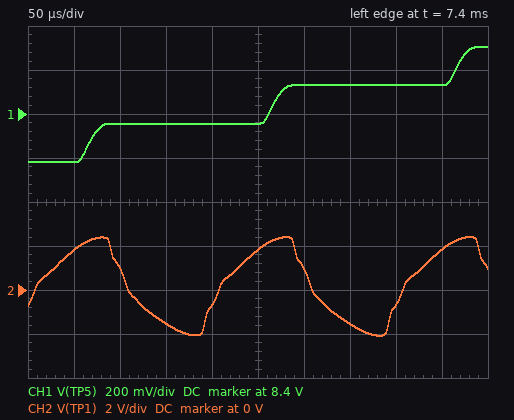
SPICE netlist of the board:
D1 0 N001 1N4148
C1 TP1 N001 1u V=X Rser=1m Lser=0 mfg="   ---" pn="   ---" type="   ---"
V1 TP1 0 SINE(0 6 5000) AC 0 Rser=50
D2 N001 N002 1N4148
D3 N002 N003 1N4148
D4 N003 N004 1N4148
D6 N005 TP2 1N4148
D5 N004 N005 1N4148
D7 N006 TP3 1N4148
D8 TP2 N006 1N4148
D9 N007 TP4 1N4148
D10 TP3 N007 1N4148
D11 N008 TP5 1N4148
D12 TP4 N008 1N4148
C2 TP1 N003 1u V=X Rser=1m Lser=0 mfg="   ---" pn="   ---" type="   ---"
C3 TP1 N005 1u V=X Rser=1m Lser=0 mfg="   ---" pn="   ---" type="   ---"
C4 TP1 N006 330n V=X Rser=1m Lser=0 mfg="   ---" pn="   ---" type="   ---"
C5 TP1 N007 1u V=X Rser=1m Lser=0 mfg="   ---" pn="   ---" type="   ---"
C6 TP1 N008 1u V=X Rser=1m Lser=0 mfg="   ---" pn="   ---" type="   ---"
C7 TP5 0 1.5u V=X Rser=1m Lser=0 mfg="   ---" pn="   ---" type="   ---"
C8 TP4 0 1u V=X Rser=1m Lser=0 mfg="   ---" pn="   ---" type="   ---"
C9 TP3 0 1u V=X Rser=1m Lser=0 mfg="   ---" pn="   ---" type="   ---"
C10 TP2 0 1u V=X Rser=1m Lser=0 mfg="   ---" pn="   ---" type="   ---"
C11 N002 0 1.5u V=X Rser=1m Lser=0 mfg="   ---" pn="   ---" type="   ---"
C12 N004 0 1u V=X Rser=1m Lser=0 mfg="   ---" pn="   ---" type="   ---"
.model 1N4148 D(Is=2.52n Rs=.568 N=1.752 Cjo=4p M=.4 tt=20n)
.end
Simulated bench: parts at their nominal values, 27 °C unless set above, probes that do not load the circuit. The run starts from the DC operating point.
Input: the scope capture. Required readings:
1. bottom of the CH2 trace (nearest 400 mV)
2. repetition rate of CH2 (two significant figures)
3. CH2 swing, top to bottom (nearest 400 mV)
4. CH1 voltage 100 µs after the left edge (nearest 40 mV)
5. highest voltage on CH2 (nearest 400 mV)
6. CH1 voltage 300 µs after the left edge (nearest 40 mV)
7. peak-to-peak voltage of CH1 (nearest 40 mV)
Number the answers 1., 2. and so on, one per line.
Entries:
1. -2.0 V
2. 5.0 kHz
3. 4.4 V
4. 8.36 V
5. 2.4 V
6. 8.52 V
7. 520 mV
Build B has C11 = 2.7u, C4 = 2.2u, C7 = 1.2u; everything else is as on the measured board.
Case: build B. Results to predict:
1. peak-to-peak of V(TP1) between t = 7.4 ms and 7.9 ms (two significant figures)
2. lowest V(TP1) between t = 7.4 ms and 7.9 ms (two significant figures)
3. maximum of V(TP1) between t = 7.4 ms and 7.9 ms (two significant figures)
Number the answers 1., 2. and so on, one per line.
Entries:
1. 4.1 V
2. -1.8 V
3. 2.3 V
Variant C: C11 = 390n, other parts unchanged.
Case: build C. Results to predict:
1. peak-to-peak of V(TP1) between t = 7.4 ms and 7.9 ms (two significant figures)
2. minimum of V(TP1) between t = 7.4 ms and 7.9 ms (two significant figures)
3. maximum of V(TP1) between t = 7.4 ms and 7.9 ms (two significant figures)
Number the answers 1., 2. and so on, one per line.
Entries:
1. 4.9 V
2. -2.3 V
3. 2.6 V
